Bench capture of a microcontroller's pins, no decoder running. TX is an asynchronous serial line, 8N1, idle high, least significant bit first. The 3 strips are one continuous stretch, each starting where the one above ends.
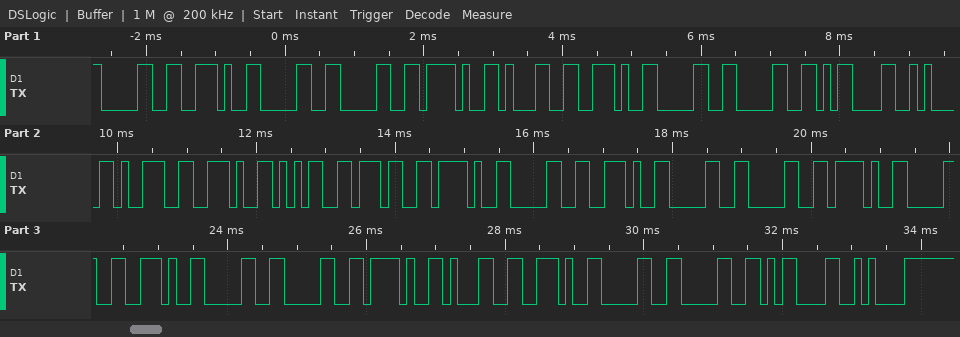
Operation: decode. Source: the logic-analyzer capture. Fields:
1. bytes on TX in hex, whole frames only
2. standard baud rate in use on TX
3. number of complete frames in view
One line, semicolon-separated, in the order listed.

30 2E 30 30 2F 31 2E 30 30 0D 0A 39 2E 35 37 2F 30 2E 30 30 2F 30 2E 30 30 2F 31 2E 30 30 0D 0A; 9600 baud; 32
